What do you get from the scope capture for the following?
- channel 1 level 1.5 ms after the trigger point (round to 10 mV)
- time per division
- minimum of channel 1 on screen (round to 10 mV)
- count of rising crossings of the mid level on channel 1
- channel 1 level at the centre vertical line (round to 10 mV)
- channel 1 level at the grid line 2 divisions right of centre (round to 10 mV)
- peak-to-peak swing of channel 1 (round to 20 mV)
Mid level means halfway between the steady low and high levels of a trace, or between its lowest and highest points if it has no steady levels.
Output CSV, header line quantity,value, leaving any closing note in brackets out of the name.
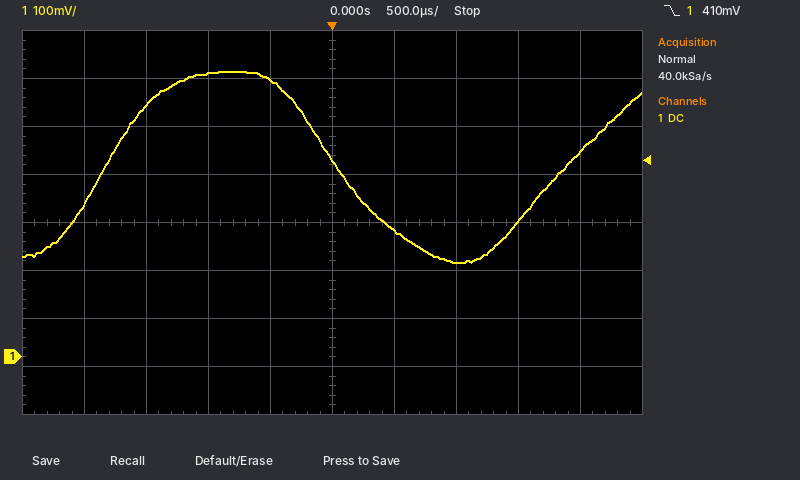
quantity,value
channel 1 level 1.5 ms after the trigger point,280 mV
time per division,500 µs
minimum of channel 1 on screen,200 mV
count of rising crossings of the mid level on channel 1,2
channel 1 level at the centre vertical line,410 mV
channel 1 level at the grid line 2 divisions right of centre,200 mV
peak-to-peak swing of channel 1,400 mV
